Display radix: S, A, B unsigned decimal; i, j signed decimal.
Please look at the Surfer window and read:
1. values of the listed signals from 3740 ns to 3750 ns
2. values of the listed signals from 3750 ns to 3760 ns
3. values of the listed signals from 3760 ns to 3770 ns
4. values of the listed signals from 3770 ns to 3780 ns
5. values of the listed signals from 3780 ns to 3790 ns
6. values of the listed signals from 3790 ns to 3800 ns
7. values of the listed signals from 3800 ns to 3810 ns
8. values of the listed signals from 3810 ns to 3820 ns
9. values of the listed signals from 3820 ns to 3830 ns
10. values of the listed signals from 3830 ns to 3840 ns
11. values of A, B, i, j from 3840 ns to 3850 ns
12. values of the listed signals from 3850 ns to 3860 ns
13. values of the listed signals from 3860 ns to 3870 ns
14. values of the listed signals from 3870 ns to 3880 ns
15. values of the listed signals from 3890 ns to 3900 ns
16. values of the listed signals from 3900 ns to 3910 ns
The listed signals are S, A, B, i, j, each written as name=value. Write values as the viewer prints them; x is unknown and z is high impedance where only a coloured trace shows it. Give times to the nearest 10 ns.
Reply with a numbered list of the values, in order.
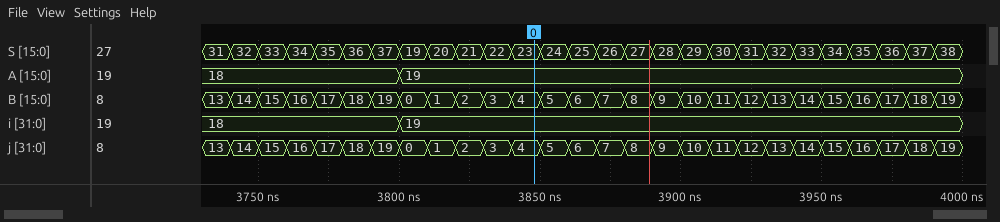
1. S=32, A=18, B=14, i=18, j=14
2. S=33, A=18, B=15, i=18, j=15
3. S=34, A=18, B=16, i=18, j=16
4. S=35, A=18, B=17, i=18, j=17
5. S=36, A=18, B=18, i=18, j=18
6. S=37, A=18, B=19, i=18, j=19
7. S=19, A=19, B=0, i=19, j=0
8. S=20, A=19, B=1, i=19, j=1
9. S=21, A=19, B=2, i=19, j=2
10. S=22, A=19, B=3, i=19, j=3
11. A=19, B=4, i=19, j=4
12. S=24, A=19, B=5, i=19, j=5
13. S=25, A=19, B=6, i=19, j=6
14. S=26, A=19, B=7, i=19, j=7
15. S=28, A=19, B=9, i=19, j=9
16. S=29, A=19, B=10, i=19, j=10
